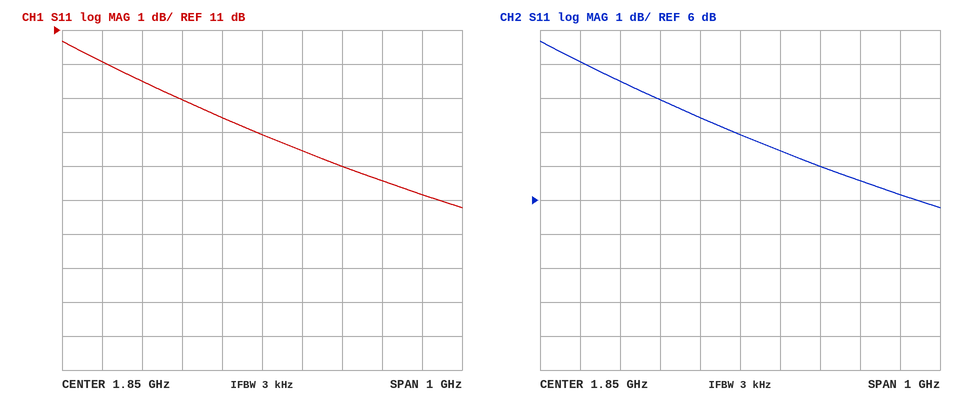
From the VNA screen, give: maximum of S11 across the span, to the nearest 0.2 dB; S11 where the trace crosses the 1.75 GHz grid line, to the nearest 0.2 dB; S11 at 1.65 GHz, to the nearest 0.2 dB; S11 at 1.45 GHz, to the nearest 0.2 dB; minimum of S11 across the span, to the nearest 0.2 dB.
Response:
10.6 dB
8.4 dB
9.0 dB
10.0 dB
5.8 dB
